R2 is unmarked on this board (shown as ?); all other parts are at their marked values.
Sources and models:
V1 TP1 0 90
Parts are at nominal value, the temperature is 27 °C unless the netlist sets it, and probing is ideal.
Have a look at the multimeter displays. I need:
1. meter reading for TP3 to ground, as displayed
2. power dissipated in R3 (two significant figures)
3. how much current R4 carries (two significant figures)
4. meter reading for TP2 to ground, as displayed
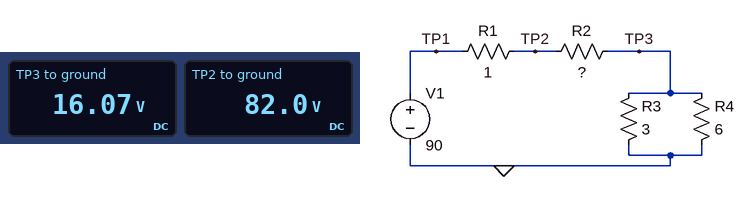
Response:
16.07 V
86 W
2.7 A
82.0 V
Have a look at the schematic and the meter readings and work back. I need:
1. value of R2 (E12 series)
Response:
8.2 Ω
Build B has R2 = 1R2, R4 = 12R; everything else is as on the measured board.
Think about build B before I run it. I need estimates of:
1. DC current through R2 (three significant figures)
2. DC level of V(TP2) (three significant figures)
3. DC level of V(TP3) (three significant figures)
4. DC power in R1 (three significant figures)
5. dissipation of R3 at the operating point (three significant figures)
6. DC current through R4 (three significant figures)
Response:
19.6 A
70.4 V
47.0 V
383 W
735 W
3.91 A
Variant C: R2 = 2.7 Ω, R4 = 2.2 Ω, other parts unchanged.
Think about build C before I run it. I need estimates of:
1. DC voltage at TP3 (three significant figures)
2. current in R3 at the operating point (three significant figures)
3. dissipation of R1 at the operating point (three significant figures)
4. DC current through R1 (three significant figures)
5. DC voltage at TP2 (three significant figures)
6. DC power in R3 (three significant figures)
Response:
23.0 V
7.66 A
328 W
18.1 A
71.9 V
176 W
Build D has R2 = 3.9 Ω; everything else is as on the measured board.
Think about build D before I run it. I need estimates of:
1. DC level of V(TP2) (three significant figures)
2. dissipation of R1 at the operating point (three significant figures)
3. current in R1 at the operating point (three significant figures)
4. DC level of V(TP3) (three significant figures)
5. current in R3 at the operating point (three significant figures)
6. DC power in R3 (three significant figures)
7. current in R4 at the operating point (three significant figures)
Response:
77.0 V
170 W
13.0 A
26.1 V
8.70 A
227 W
4.35 A
